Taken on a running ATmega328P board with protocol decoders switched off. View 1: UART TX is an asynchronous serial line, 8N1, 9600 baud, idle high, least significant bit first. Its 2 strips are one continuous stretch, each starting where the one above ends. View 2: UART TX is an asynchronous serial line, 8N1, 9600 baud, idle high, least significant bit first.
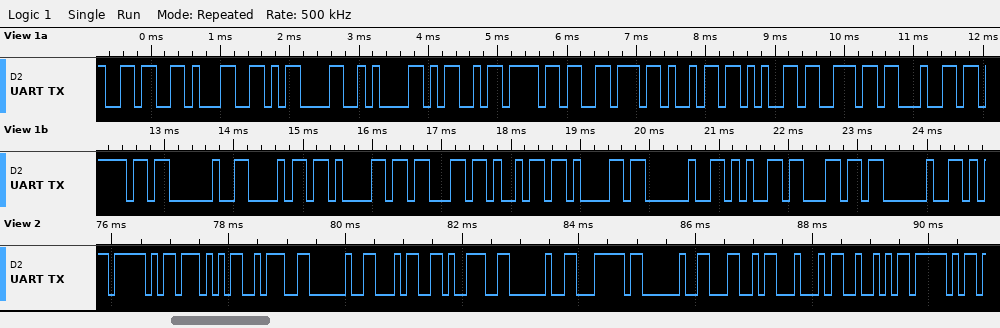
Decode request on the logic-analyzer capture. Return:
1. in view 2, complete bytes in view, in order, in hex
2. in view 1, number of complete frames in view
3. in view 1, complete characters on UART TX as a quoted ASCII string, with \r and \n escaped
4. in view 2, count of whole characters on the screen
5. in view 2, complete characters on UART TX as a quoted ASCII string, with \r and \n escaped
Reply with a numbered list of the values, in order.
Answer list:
1. 5F 57 3A 20 34 39 20 7C 20 4C 44 52 5F
2. 22
3. "61\r\nMoviendo hacia el "
4. 13
5. "_W: 49 | LDR_"
